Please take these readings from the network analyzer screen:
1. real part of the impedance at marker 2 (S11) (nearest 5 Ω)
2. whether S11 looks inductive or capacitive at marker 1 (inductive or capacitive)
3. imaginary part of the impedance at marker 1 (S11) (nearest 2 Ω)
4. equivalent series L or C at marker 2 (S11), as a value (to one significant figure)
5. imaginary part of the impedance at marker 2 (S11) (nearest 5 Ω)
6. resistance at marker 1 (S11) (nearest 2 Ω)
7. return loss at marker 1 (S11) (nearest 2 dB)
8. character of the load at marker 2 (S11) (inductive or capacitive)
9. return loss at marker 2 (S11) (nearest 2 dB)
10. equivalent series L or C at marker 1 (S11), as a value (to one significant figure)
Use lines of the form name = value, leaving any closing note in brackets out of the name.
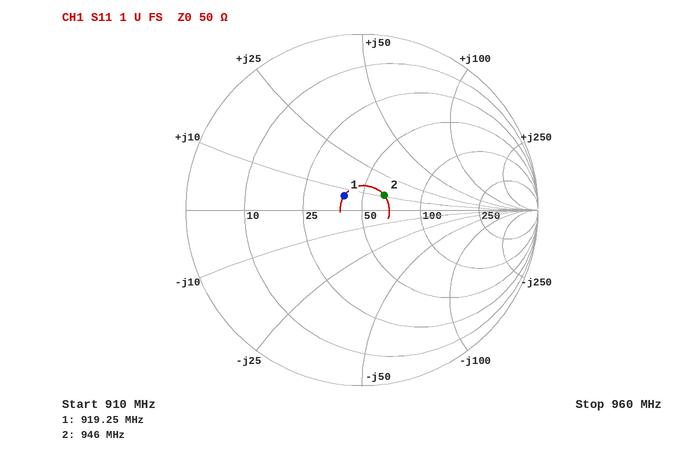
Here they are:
real part of the impedance at marker 2 (S11) = 65 Ω
whether S11 looks inductive or capacitive at marker 1 = inductive
imaginary part of the impedance at marker 1 (S11) = +6 Ω
equivalent series L or C at marker 2 (S11), as a value = 2 nH
imaginary part of the impedance at marker 2 (S11) = +10 Ω
resistance at marker 1 (S11) = 40 Ω
return loss at marker 1 (S11) = 18 dB
character of the load at marker 2 (S11) = inductive
return loss at marker 2 (S11) = 16 dB
equivalent series L or C at marker 1 (S11), as a value = 1 nH
